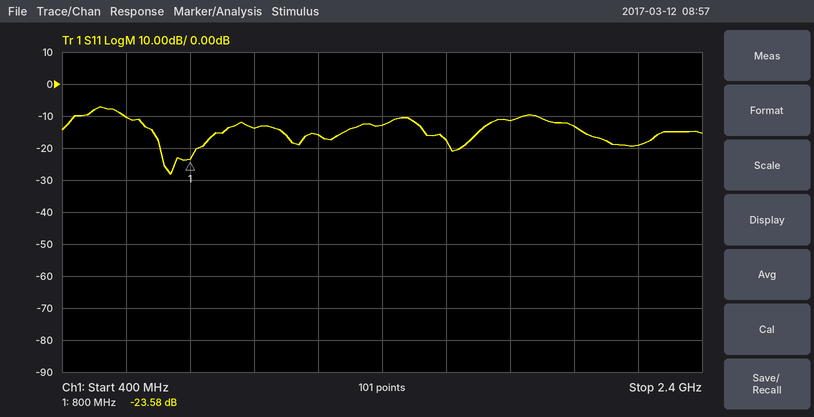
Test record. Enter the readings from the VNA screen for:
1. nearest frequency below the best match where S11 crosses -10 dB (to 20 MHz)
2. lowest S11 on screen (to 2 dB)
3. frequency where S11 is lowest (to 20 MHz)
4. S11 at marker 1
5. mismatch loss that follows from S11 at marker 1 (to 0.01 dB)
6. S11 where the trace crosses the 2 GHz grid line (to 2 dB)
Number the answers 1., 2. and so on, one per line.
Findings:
1. 600 MHz
2. -28 dB
3. 740 MHz
4. -23.58 dB
5. 0.02 dB
6. -14 dB
